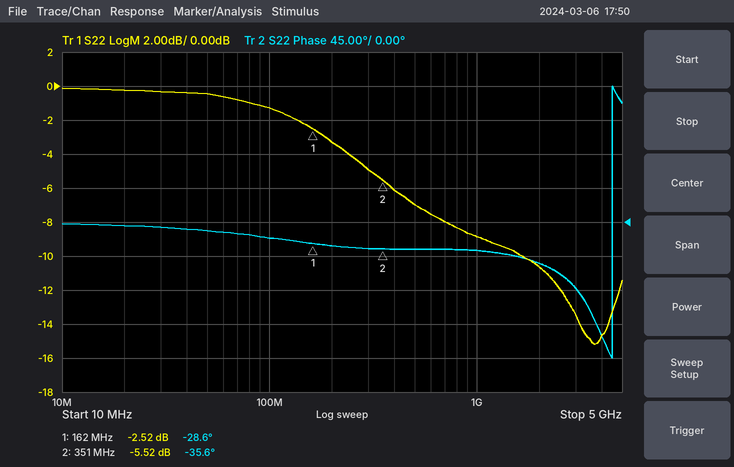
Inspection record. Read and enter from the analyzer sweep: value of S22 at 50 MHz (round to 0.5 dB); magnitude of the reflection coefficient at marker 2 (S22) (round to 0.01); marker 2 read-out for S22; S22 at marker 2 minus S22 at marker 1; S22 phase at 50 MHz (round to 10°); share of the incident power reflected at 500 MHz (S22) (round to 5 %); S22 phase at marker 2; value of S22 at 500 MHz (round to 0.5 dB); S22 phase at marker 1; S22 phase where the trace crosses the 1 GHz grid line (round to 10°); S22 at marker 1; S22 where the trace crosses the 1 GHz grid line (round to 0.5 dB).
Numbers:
-0.5 dB
0.53
-5.52 dB
-3.00 dB
-10°
20 %
-35.6°
-7.0 dB
-28.6°
-40°
-2.52 dB
-9.0 dB
